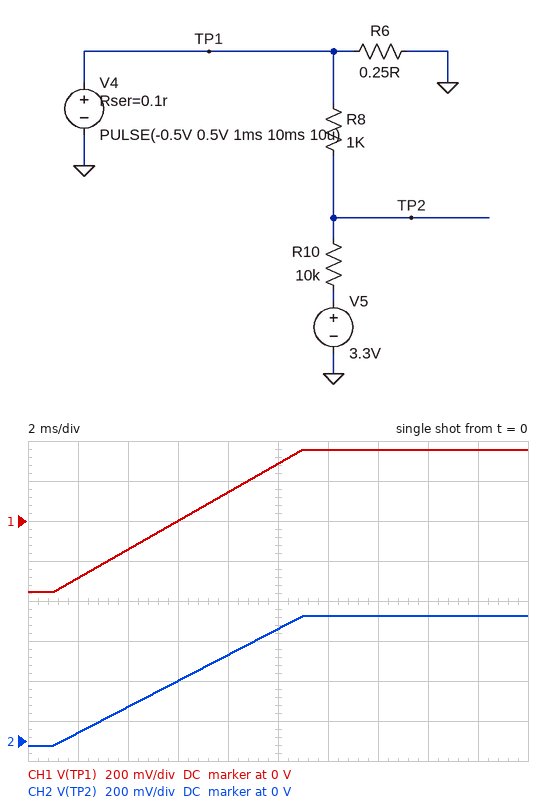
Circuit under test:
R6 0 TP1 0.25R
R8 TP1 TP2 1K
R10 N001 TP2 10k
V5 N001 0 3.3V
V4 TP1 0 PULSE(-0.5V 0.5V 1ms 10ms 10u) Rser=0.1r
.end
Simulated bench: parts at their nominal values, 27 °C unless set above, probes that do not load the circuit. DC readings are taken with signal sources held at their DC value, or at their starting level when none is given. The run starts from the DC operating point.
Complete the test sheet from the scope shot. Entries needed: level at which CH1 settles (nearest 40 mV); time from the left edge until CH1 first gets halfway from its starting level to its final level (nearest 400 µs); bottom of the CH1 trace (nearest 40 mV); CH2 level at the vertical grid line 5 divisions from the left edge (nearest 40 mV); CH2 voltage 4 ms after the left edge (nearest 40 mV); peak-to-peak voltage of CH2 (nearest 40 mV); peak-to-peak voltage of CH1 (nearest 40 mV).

360 mV
6.0 ms
-360 mV
560 mV
160 mV
640 mV
720 mV
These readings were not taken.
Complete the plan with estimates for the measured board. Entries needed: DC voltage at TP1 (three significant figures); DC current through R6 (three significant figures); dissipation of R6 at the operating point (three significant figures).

-357 mV
1.43 A
510 mW
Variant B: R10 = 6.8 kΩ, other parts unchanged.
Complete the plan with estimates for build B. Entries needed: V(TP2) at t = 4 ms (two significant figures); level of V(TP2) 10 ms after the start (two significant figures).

300 mV
670 mV
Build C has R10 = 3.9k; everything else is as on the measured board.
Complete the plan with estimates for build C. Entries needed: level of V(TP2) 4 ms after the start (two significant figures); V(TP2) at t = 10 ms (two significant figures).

560 mV
900 mV
